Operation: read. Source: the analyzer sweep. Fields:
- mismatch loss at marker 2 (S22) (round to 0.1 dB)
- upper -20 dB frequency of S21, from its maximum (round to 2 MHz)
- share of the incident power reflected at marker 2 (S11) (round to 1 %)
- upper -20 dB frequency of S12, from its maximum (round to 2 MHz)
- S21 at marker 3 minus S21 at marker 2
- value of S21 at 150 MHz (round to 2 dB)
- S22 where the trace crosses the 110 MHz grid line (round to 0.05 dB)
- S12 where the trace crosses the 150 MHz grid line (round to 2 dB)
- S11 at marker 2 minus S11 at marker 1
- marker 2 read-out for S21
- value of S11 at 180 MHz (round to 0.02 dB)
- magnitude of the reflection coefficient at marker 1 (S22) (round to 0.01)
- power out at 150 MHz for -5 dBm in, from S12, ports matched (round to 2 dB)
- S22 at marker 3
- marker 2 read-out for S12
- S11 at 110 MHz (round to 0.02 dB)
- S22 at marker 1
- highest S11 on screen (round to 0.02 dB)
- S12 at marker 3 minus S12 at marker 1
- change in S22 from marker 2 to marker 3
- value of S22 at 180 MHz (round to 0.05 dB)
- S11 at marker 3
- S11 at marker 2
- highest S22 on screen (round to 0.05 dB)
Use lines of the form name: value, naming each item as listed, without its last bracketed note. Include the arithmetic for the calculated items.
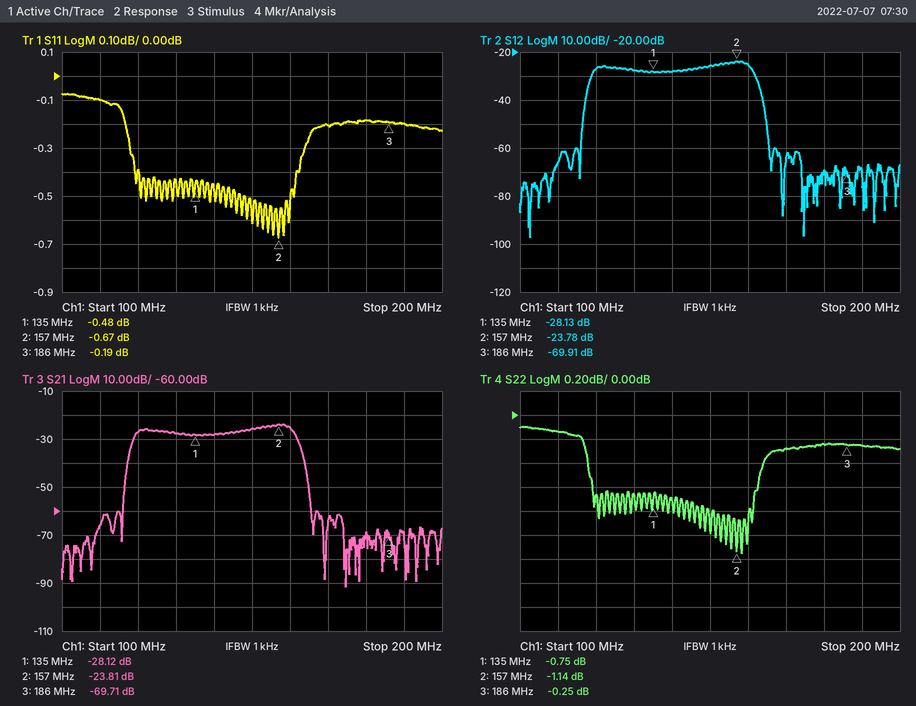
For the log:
mismatch loss at marker 2 (S22): −10 log10(1 − 10^(-1.14/10)) ≈ 6.4 dB
upper -20 dB frequency of S21, from its maximum: 164 MHz
share of the incident power reflected at marker 2 (S11): 10^(-0.67/10) ≈ 86 %
upper -20 dB frequency of S12, from its maximum: 164 MHz
S21 at marker 3 minus S21 at marker 2: -69.71 − (-23.81) = -45.90 dB
value of S21 at 150 MHz: -26 dB
S22 where the trace crosses the 110 MHz grid line: -0.15 dB
S12 where the trace crosses the 150 MHz grid line: -26 dB
S11 at marker 2 minus S11 at marker 1: -0.67 − (-0.48) = -0.19 dB
marker 2 read-out for S21: -23.81 dB
value of S11 at 180 MHz: -0.18 dB
magnitude of the reflection coefficient at marker 1 (S22): 10^(-0.75/20) ≈ 0.92
power out at 150 MHz for -5 dBm in, from S12, ports matched: -5 dBm + (-26 dB) = -30 dBm
S22 at marker 3: -0.25 dB
marker 2 read-out for S12: -23.78 dB
S11 at 110 MHz: -0.10 dB
S22 at marker 1: -0.75 dB
highest S11 on screen: -0.08 dB
S12 at marker 3 minus S12 at marker 1: -69.91 − (-28.13) = -41.78 dB
change in S22 from marker 2 to marker 3: -0.25 − (-1.14) = 0.89 dB
value of S22 at 180 MHz: -0.25 dB
S11 at marker 3: -0.19 dB
S11 at marker 2: -0.67 dB
highest S22 on screen: -0.10 dB
